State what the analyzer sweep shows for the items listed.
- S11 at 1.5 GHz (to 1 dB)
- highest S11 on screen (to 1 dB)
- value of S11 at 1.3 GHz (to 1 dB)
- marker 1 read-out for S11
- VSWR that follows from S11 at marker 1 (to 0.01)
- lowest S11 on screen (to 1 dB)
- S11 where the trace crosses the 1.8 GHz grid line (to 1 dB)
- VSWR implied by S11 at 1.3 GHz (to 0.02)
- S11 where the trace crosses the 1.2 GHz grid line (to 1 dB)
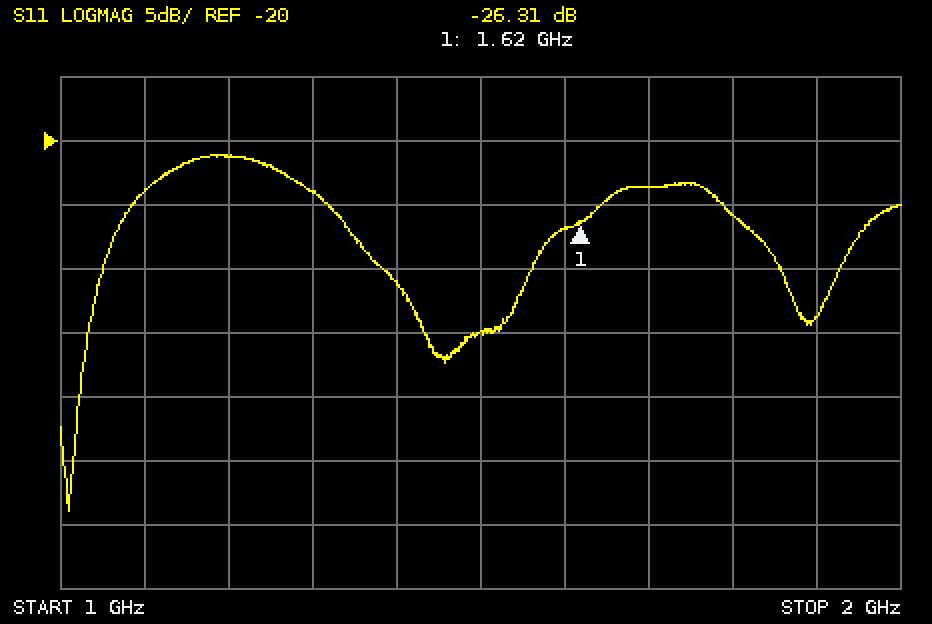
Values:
-35 dB
-21 dB
-24 dB
-26.31 dB
1.10
-49 dB
-26 dB
1.14
-21 dB
